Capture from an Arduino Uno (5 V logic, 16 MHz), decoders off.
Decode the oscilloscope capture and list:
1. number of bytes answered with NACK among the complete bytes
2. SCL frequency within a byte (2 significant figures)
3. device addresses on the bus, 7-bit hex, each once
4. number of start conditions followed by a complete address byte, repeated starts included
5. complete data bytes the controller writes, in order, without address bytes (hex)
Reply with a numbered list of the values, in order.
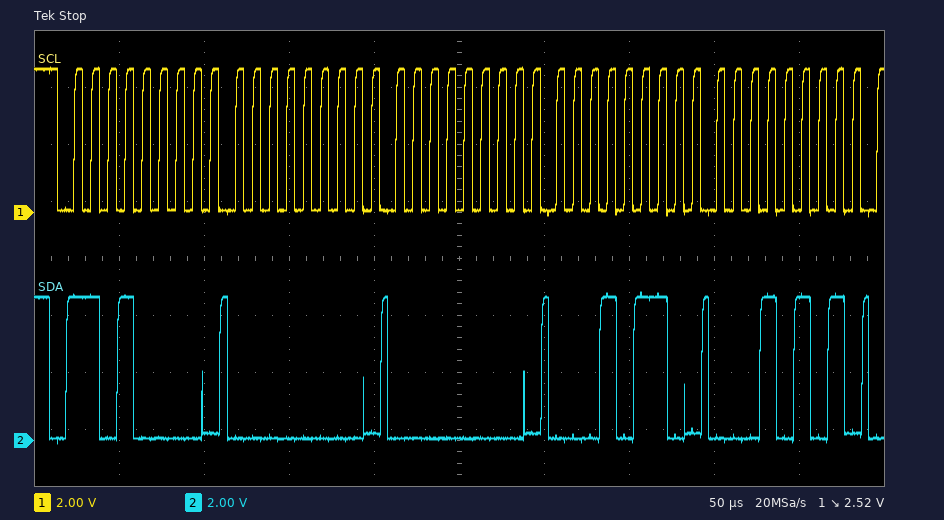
1. 0
2. 100 kHz
3. 0x68
4. 1
5. 00 00 16 15
